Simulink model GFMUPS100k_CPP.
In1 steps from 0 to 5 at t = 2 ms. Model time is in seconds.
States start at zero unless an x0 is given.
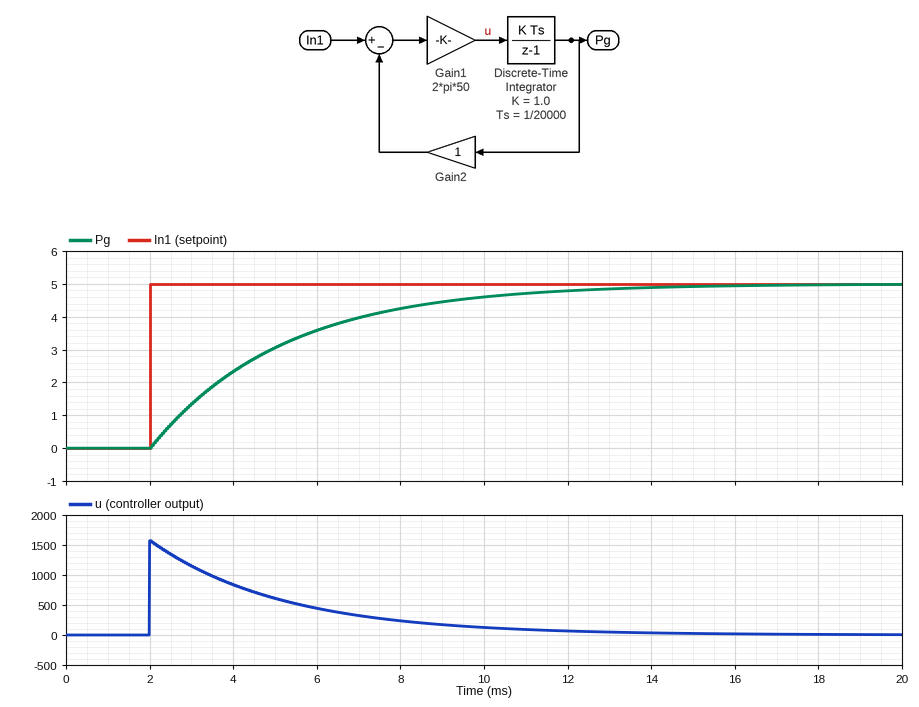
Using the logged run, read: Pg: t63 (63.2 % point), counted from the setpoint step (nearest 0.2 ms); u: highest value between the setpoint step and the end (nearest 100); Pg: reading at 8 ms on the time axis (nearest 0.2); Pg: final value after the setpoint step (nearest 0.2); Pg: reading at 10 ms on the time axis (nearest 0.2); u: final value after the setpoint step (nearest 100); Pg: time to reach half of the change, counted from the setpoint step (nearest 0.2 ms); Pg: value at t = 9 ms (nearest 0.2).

3.2 ms
1600
4.2
5.0
4.6
0
2.2 ms
4.4
